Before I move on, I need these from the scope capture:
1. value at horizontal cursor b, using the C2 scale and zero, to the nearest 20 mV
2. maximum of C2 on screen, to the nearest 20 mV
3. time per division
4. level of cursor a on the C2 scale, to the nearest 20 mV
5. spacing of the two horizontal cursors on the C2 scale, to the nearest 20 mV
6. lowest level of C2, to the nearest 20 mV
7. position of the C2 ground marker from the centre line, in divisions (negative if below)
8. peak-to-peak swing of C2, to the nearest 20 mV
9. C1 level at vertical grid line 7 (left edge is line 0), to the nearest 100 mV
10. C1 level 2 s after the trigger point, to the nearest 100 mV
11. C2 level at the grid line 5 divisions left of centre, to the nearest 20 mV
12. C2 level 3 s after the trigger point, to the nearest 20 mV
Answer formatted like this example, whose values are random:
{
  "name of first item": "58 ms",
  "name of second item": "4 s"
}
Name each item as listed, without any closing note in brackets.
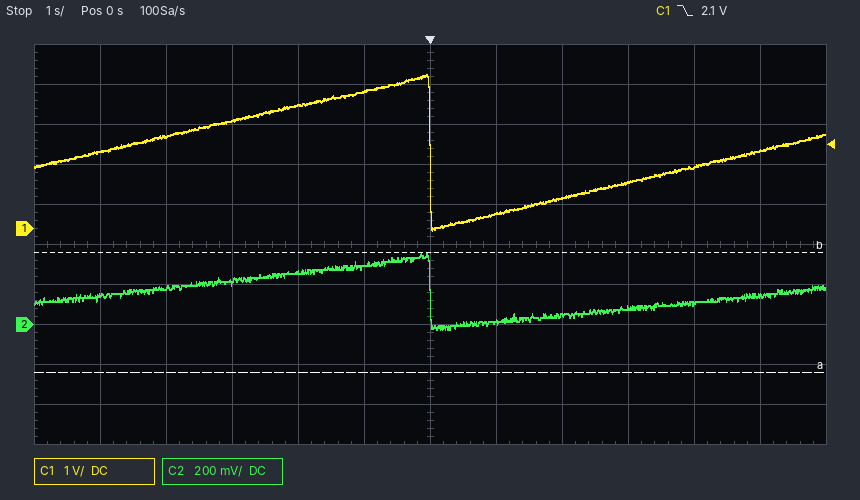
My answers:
{
  "value at horizontal cursor b, using the C2 scale and zero, to the nearest 20 mV": "360 mV",
  "maximum of C2 on screen, to the nearest 20 mV": "360 mV",
  "time per division": "1 s",
  "level of cursor a on the C2 scale, to the nearest 20 mV": "-240 mV",
  "spacing of the two horizontal cursors on the C2 scale, to the nearest 20 mV": "600 mV",
  "lowest level of C2, to the nearest 20 mV": "-20 mV",
  "position of the C2 ground marker from the centre line, in divisions": "-2.0 div",
  "peak-to-peak swing of C2, to the nearest 20 mV": "380 mV",
  "C1 level at vertical grid line 7 (left edge is line 0), to the nearest 100 mV": "400 mV",
  "C1 level 2 s after the trigger point, to the nearest 100 mV": "800 mV",
  "C2 level at the grid line 5 divisions left of centre, to the nearest 20 mV": "140 mV",
  "C2 level 3 s after the trigger point, to the nearest 20 mV": "80 mV"
}
